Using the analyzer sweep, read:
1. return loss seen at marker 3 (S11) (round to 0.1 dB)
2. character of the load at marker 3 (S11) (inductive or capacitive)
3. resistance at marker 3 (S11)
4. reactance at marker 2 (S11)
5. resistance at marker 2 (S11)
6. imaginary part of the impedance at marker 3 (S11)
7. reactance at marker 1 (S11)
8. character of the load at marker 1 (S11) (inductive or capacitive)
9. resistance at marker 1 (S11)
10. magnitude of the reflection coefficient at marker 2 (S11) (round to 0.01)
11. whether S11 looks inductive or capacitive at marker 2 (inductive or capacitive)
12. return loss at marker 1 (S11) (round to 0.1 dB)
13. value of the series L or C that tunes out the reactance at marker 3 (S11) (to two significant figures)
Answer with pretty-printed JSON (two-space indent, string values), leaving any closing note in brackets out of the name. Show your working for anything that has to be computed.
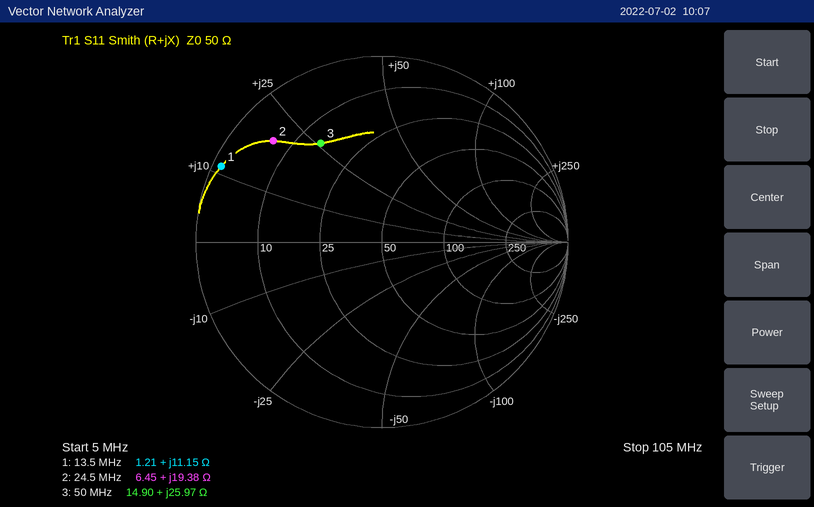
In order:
{
  "return loss seen at marker 3 (S11)": "4.1 dB",
  "character of the load at marker 3 (S11)": "inductive",
  "resistance at marker 3": "14.90 Ω",
  "reactance at marker 2": "+19.38 Ω",
  "resistance at marker 2": "6.45 Ω",
  "imaginary part of the impedance at marker 3": "+25.97 Ω",
  "reactance at marker 1": "+11.15 Ω",
  "character of the load at marker 1 (S11)": "inductive",
  "resistance at marker 1": "1.21 Ω",
  "magnitude of the reflection coefficient at marker 2 (S11)": "0.80",
  "whether S11 looks inductive or capacitive at marker 2": "inductive",
  "return loss at marker 1 (S11)": "0.4 dB",
  "value of the series L or C that tunes out the reactance at marker 3 (S11)": "C = 1/(2π × 50 MHz × 25.97 Ω) ≈ 123 pF, so 120 pF to two significant figures"
}
